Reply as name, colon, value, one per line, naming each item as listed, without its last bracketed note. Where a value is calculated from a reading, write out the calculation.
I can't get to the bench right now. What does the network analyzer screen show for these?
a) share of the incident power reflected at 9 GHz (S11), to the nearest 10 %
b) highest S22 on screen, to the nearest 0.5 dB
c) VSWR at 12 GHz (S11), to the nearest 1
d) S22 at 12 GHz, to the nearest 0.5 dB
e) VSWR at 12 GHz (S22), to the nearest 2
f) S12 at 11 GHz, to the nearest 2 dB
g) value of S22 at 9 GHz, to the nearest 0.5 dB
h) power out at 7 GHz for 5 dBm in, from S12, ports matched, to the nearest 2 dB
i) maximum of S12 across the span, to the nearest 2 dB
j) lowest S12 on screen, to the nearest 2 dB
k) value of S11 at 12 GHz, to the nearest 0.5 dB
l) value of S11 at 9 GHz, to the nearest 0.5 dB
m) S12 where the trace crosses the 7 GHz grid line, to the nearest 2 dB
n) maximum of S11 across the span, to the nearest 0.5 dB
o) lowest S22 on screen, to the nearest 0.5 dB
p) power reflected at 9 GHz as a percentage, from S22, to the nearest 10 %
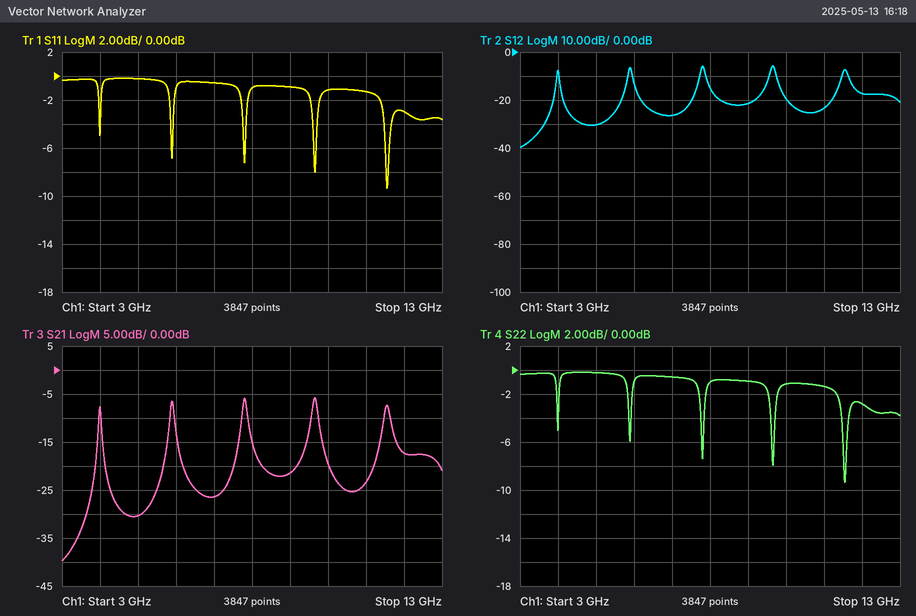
share of the incident power reflected at 9 GHz (S11), to the nearest 10 %: 10^(-1/10) ≈ 79.4 %, so 80 % to the nearest 10 %
highest S22 on screen, to the nearest 0.5 dB: 0.0 dB
VSWR at 12 GHz (S11), to the nearest 1: |Γ| = 10^(-3/20) = 0.7079; VSWR = (1 + 0.7079)/(1 − 0.7079) ≈ 6
S22 at 12 GHz, to the nearest 0.5 dB: -3.0 dB
VSWR at 12 GHz (S22), to the nearest 2: |Γ| = 10^(-3/20) = 0.7079; VSWR = (1 + 0.7079)/(1 − 0.7079) ≈ 6
S12 at 11 GHz, to the nearest 2 dB: -24 dB
value of S22 at 9 GHz, to the nearest 0.5 dB: -1.0 dB
power out at 7 GHz for 5 dBm in, from S12, ports matched, to the nearest 2 dB: 5 dBm + (-26 dB) = -22 dBm
maximum of S12 across the span, to the nearest 2 dB: -6 dB
lowest S12 on screen, to the nearest 2 dB: -40 dB
value of S11 at 12 GHz, to the nearest 0.5 dB: -3.0 dB
value of S11 at 9 GHz, to the nearest 0.5 dB: -1.0 dB
S12 where the trace crosses the 7 GHz grid line, to the nearest 2 dB: -26 dB
maximum of S11 across the span, to the nearest 0.5 dB: 0.0 dB
lowest S22 on screen, to the nearest 0.5 dB: -9.5 dB
power reflected at 9 GHz as a percentage, from S22, to the nearest 10 %: 10^(-1/10) ≈ 79.4 %, so 80 % to the nearest 10 %
